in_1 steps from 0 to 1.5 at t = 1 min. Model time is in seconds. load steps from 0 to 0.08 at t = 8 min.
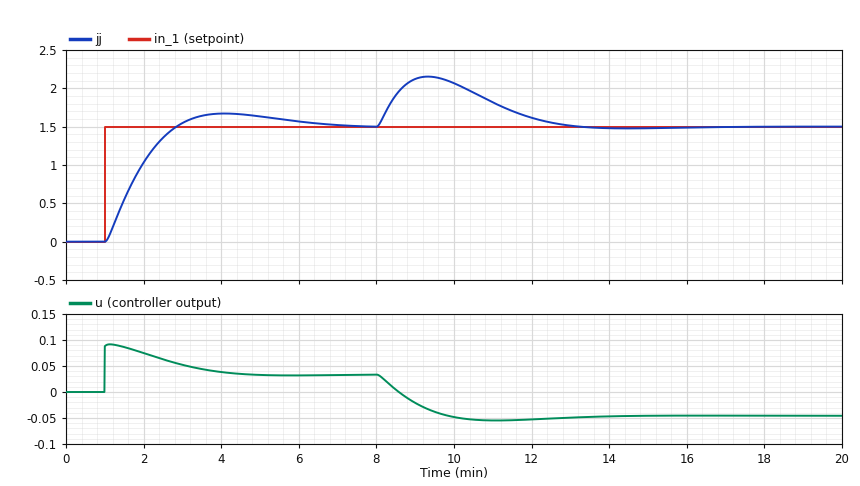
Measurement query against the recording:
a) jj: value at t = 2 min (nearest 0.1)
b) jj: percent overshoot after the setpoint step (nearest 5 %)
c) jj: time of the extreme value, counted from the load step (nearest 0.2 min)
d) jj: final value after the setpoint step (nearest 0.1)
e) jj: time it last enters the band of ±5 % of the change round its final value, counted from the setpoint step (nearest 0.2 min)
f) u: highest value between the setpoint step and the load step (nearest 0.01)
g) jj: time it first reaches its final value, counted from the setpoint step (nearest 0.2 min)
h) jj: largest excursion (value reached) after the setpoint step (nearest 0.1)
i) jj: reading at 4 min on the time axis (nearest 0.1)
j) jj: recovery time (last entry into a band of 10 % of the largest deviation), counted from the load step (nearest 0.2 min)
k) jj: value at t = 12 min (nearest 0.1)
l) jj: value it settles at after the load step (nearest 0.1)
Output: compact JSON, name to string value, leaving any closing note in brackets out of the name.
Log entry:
{"jj: value at t = 2 min": "1.0", "jj: percent overshoot after the setpoint step": "10 %", "jj: time of the extreme value, counted from the load step": "1.4 min", "jj: final value after the setpoint step": "1.5", "jj: time it last enters the band of ±5 % of the change round its final value, counted from the setpoint step": "4.8 min", "u: highest value between the setpoint step and the load step": "0.09", "jj: time it first reaches its final value, counted from the setpoint step": "1.8 min", "jj: largest excursion (value reached) after the setpoint step": "1.7", "jj: reading at 4 min on the time axis": "1.7", "jj: recovery time (last entry into a band of 10 % of the largest deviation), counted from the load step": "4.4 min", "jj: value at t = 12 min": "1.6", "jj: value it settles at after the load step": "1.5"}
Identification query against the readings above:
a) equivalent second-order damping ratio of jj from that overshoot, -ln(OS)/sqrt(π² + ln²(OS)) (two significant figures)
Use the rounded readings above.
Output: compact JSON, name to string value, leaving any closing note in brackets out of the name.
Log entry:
{"equivalent second-order damping ratio of jj from that overshoot, -ln(OS)/sqrt(π² + ln²(OS))": "0.59"}
